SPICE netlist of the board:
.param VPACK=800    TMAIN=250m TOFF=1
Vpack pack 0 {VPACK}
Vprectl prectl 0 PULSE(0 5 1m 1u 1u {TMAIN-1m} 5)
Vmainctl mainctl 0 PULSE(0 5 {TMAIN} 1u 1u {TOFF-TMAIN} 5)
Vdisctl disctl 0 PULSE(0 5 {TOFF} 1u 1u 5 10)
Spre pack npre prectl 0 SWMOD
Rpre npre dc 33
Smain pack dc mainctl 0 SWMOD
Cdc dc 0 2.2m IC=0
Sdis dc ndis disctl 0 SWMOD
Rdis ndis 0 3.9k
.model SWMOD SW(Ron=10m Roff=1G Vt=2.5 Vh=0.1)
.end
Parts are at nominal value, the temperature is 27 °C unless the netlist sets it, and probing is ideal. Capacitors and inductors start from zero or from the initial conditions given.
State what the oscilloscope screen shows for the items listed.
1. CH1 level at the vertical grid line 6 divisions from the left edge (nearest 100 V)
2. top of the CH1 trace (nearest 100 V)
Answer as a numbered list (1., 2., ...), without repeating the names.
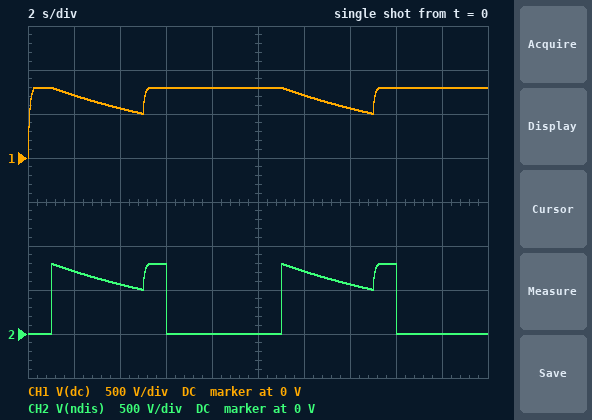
1. 700 V
2. 800 V
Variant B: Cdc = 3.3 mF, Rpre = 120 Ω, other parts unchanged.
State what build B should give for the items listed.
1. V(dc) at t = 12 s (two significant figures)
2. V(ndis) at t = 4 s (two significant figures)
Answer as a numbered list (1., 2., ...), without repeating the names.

1. 740 V
2. 630 V
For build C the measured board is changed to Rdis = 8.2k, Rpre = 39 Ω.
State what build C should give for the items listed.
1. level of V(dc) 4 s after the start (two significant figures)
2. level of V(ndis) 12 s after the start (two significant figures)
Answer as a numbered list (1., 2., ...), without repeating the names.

1. 680 V
2. 760 V
